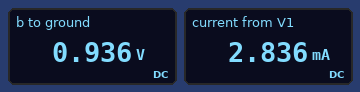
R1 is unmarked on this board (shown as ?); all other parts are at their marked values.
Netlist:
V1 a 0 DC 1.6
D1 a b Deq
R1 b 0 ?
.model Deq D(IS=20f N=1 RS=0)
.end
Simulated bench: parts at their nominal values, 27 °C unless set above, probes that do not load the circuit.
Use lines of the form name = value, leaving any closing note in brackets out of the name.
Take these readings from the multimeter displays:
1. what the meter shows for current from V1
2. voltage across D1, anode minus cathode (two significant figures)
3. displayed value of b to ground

what the meter shows for current from V1 = 2.836 mA
voltage across D1, anode minus cathode = 660 mV
displayed value of b to ground = 0.936 V
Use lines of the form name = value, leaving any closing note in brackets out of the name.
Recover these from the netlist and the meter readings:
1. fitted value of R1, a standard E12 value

fitted value of R1, a standard E12 value = 330 Ω
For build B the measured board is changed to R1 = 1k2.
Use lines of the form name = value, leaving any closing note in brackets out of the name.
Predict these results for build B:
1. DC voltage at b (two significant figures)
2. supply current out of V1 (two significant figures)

DC voltage at b = 970 mV
supply current out of V1 = 810 µA
